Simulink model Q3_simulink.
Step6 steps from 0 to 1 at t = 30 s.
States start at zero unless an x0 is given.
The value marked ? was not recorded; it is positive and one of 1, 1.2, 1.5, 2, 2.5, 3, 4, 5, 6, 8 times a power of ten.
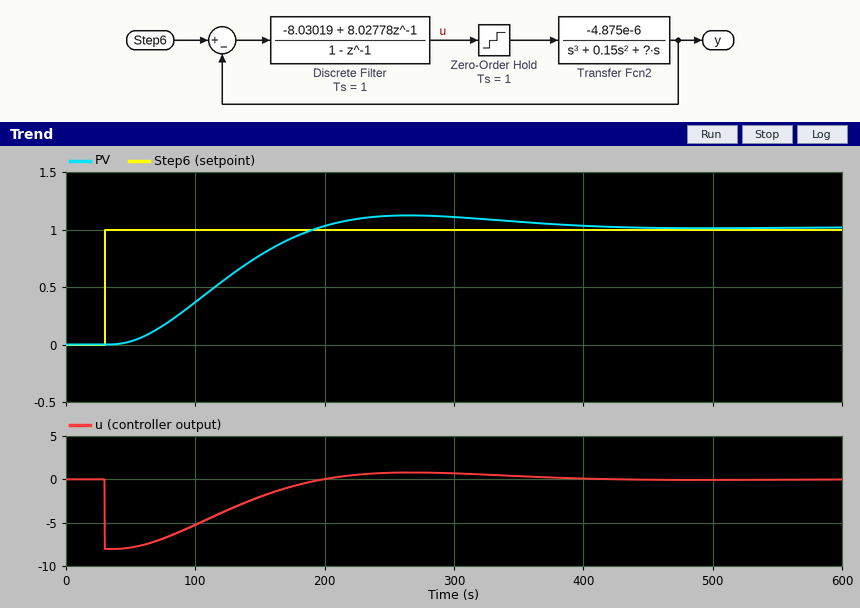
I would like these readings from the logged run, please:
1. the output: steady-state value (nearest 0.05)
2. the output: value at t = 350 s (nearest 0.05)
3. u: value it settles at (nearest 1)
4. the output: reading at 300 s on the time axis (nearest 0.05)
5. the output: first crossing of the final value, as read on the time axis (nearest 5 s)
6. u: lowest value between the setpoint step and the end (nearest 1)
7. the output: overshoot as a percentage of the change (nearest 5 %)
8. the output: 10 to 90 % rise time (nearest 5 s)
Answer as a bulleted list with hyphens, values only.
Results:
- 1.00
- 1.05
- 0
- 1.10
- 195 s
- -8
- 10 %
- 105 s
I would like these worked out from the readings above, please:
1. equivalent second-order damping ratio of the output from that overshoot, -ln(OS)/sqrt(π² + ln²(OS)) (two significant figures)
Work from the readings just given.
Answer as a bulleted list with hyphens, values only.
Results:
- 0.59
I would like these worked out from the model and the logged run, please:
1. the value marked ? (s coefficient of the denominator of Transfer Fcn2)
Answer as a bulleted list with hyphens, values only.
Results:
- 0.003
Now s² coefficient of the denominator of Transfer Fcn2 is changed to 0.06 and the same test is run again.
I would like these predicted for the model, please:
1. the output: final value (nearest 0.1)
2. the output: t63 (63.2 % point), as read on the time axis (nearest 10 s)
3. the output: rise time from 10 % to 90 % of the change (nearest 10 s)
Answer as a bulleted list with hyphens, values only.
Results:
- 1.0
- 110 s
- 100 s
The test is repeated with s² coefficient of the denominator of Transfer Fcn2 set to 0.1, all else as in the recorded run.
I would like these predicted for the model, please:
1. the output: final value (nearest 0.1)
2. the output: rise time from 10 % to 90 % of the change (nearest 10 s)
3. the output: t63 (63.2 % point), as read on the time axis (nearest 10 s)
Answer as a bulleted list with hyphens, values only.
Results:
- 1.0
- 100 s
- 120 s
